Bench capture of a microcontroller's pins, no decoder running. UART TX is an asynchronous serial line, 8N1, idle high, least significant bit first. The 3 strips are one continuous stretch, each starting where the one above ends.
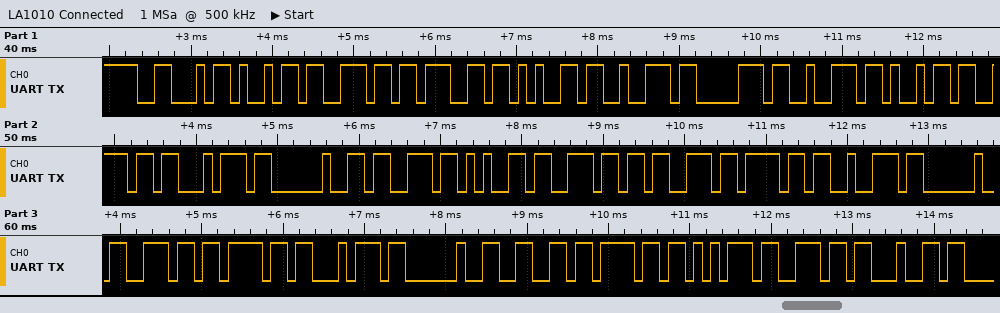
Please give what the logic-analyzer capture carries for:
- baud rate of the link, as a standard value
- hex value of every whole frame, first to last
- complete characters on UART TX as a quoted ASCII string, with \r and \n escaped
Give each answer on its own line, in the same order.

9600 baud
46 69 6E 67 65 72 70 72 69 6E 74 20 73 65 6E 73 6F 72 20 6E 6F 74 20 66 6F 75 6E 64
"Fingerprint sensor not found"
